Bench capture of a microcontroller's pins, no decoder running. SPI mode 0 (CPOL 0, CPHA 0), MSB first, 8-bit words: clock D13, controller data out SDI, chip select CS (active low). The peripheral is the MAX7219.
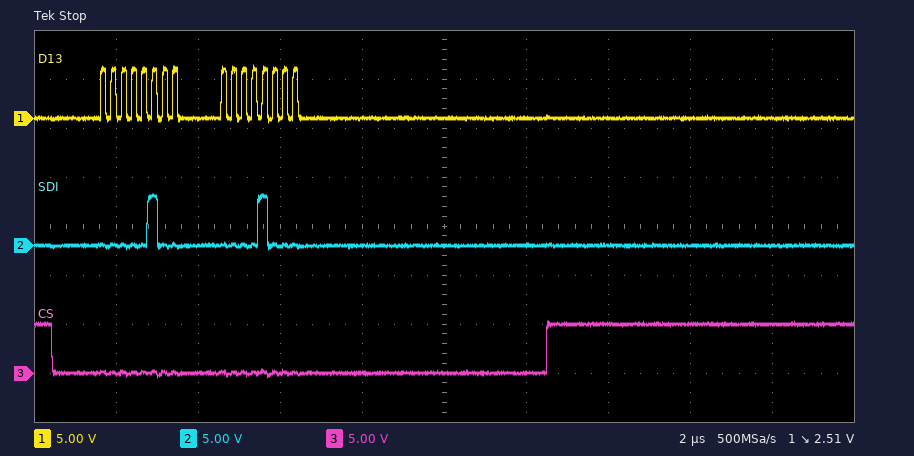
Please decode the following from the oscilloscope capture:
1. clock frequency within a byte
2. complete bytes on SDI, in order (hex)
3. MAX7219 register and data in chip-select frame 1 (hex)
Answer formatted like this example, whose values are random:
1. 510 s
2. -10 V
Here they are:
1. 4 MHz
2. 04 08
3. register 0x4, data 0x08
